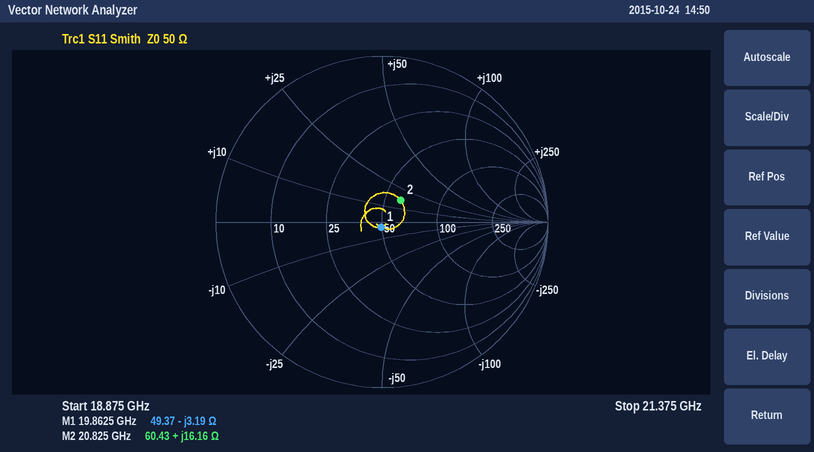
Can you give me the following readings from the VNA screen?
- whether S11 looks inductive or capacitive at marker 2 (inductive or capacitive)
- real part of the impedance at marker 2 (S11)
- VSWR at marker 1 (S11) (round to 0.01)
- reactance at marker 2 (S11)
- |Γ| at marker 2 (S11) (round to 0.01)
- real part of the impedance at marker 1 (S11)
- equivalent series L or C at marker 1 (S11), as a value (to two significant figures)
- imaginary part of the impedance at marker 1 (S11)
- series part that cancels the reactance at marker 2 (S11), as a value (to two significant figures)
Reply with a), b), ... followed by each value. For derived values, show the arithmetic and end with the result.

a) inductive
b) 60.43 Ω
c) 1.07
d) +16.16 Ω
e) 0.17
f) 49.37 Ω
g) C = 1/(2π × 19.8625 GHz × 3.19 Ω) ≈ 2.5 pF
h) -3.19 Ω
i) C = 1/(2π × 20.825 GHz × 16.16 Ω) ≈ 473 fF, so 470 fF to two significant figures
